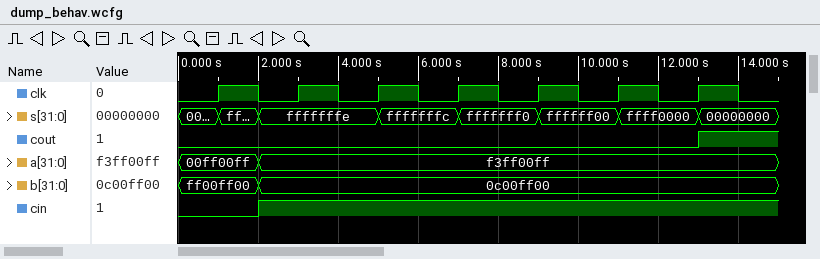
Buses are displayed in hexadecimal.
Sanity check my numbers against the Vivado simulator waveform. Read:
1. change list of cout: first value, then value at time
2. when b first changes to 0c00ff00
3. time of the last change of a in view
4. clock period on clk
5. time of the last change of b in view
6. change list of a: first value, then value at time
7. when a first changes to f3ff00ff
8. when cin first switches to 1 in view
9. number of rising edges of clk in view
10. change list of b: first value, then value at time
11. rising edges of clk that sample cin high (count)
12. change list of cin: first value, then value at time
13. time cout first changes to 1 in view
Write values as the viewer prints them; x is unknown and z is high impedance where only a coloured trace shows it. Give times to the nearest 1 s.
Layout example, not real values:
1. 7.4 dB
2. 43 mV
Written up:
1. 0, 1 at 13 s
2. 2 s
3. 2 s
4. 2 s
5. 2 s
6. 00ff00ff, f3ff00ff at 2 s
7. 2 s
8. 2 s
9. 7
10. ff00ff00, 0c00ff00 at 2 s
11. 6
12. 0, 1 at 2 s
13. 13 s
